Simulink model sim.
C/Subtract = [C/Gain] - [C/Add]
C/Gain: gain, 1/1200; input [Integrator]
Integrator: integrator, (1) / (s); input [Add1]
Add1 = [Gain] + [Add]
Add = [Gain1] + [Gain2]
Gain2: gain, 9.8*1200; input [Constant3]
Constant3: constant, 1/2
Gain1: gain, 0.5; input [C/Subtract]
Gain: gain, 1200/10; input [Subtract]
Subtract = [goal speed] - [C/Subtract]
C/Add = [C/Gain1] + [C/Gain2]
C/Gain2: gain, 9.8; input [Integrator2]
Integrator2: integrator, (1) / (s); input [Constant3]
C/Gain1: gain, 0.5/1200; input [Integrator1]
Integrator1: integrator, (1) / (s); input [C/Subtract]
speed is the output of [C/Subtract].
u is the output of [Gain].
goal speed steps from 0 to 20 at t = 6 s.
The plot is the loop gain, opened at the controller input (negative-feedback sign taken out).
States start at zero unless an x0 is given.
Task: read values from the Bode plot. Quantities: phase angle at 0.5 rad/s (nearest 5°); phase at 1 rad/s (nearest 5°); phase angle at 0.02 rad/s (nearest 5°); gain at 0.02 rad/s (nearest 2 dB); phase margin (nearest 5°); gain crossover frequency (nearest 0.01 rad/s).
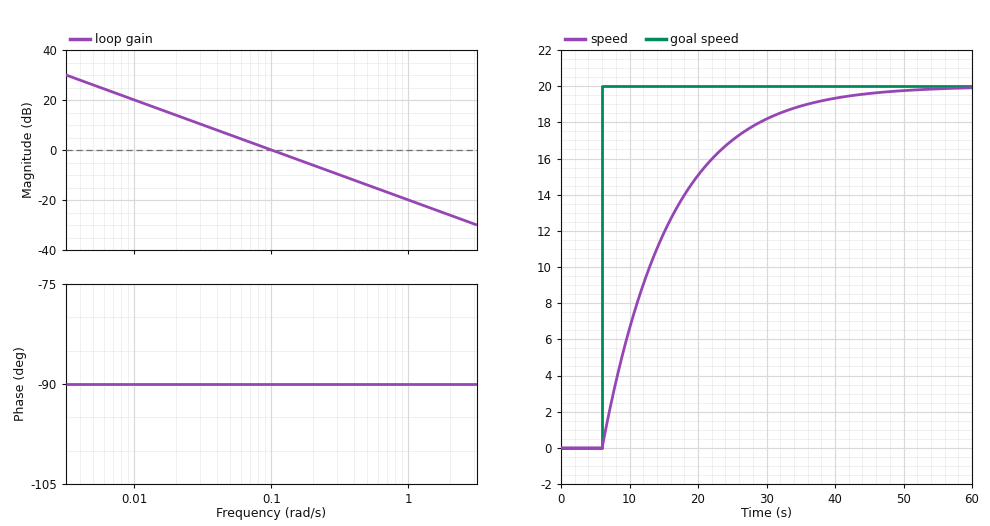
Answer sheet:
-90°
-90°
-90°
14 dB
90°
0.10 rad/s
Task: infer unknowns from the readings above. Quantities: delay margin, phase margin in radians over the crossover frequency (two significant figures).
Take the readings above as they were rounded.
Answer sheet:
16 s
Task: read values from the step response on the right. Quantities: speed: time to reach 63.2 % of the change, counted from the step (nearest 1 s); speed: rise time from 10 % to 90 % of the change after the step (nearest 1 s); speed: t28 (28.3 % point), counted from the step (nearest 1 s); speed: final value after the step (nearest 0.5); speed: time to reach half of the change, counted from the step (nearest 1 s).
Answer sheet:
10 s
22 s
3 s
20.0
7 s
